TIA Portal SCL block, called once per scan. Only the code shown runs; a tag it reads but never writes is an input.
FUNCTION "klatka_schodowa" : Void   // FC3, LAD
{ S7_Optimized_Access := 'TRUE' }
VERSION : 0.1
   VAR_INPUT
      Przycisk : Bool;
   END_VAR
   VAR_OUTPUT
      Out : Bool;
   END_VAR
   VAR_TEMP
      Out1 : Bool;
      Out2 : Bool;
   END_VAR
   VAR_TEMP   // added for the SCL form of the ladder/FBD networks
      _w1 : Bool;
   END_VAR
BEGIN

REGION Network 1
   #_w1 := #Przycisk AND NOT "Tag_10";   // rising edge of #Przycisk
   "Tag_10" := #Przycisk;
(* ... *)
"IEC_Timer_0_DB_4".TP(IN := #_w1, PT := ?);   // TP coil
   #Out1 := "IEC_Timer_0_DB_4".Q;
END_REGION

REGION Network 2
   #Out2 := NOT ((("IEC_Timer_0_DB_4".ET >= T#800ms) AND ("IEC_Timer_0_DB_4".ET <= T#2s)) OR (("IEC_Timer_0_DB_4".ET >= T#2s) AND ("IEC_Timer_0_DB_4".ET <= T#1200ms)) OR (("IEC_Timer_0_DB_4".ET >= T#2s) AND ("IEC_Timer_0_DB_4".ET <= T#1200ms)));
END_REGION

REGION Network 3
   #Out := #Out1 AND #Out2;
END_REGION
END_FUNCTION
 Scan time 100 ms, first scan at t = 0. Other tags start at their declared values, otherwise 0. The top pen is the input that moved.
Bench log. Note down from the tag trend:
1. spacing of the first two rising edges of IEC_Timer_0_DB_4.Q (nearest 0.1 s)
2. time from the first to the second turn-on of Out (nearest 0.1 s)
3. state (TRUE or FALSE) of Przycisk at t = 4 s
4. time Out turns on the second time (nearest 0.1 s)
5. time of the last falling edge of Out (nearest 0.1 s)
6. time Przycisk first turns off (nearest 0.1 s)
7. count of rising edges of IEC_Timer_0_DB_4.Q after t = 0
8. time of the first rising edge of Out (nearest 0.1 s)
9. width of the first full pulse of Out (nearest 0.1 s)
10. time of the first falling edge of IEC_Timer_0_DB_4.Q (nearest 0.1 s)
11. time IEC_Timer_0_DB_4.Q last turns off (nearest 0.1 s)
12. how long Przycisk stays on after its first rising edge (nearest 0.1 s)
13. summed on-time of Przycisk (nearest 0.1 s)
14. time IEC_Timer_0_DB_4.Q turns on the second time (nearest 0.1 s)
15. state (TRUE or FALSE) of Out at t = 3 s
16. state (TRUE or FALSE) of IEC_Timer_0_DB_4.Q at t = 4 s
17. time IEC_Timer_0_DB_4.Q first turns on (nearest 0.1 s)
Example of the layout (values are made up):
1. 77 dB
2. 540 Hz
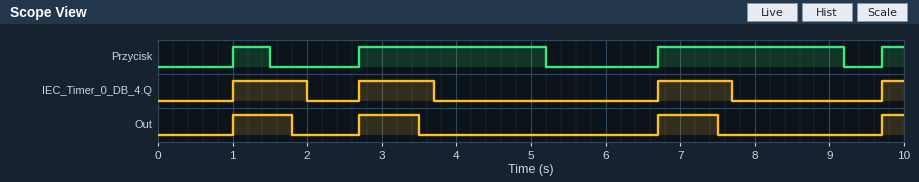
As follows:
1. 1.7 s
2. 1.7 s
3. TRUE
4. 2.7 s
5. 7.5 s
6. 1.5 s
7. 4
8. 1.0 s
9. 0.8 s
10. 2.0 s
11. 7.7 s
12. 0.5 s
13. 5.8 s
14. 2.7 s
15. TRUE
16. FALSE
17. 1.0 s
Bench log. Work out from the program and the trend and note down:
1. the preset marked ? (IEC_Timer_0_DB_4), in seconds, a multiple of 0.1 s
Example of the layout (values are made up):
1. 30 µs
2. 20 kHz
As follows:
1. 1.0 s
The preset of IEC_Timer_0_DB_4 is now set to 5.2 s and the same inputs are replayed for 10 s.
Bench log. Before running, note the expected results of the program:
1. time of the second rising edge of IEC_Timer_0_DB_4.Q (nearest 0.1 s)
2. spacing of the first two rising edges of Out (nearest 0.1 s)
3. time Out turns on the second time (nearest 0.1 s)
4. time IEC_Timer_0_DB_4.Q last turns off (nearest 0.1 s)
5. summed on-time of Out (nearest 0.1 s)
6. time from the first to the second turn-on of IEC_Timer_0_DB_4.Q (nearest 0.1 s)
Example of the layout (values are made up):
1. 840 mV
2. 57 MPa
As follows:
1. 6.7 s
2. 2.1 s
3. 3.1 s
4. 6.2 s
5. 5.9 s
6. 5.7 s
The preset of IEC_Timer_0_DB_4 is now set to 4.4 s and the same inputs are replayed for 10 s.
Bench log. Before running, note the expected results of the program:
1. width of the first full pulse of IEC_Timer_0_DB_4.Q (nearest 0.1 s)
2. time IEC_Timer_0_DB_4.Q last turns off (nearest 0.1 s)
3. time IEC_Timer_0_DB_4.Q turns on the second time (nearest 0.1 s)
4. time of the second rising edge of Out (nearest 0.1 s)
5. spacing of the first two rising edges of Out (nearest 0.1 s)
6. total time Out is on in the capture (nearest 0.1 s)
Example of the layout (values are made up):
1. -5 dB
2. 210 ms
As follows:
1. 4.4 s
2. 5.4 s
3. 6.7 s
4. 3.1 s
5. 2.1 s
6. 5.1 s
